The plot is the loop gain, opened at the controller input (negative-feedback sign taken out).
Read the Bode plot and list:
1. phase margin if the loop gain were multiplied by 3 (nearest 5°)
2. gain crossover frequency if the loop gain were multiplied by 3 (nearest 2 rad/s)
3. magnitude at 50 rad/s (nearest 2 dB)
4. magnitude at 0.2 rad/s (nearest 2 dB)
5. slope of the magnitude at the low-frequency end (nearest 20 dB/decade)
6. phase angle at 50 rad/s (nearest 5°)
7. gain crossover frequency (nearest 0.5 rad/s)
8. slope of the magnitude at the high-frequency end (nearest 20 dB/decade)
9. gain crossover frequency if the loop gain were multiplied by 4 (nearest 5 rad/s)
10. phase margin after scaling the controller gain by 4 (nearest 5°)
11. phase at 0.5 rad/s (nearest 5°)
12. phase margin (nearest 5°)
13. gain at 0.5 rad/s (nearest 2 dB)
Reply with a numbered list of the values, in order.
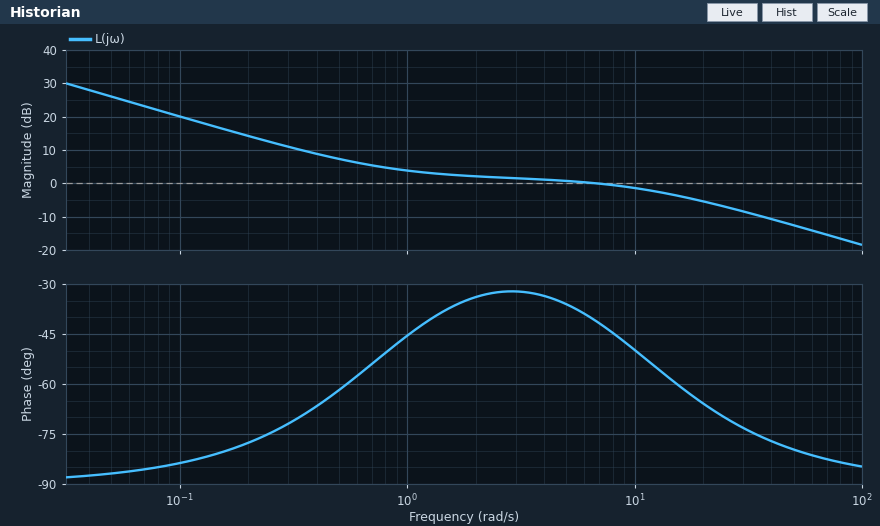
1. 105°
2. 34 rad/s
3. -12 dB
4. 14 dB
5. -20 dB/decade
6. -80°
7. 7.0 rad/s
8. -20 dB/decade
9. 45 rad/s
10. 100°
11. -60°
12. 140°
13. 8 dB
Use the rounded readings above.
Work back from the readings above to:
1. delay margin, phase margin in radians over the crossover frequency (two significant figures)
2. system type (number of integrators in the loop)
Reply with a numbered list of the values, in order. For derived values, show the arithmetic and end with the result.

1. 140 × π / 180 / 7 = 0.35 s
2. 1
